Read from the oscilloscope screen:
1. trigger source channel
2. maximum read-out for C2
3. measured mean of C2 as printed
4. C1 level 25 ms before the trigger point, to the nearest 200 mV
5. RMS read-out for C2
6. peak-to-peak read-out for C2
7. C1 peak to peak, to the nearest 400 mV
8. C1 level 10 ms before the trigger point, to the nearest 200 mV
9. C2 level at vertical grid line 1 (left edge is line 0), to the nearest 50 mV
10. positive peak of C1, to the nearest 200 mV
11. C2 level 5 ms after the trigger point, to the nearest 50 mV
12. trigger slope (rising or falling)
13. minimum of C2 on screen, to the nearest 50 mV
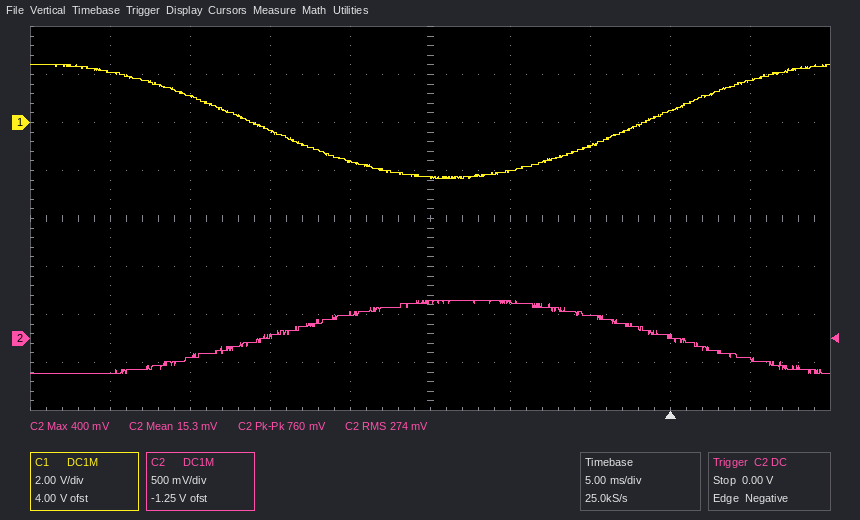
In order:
C2
400 mV
15.3 mV
-400 mV
274 mV
760 mV
4.8 V
-2.0 V
-350 mV
2.4 V
-200 mV
falling
-350 mV
